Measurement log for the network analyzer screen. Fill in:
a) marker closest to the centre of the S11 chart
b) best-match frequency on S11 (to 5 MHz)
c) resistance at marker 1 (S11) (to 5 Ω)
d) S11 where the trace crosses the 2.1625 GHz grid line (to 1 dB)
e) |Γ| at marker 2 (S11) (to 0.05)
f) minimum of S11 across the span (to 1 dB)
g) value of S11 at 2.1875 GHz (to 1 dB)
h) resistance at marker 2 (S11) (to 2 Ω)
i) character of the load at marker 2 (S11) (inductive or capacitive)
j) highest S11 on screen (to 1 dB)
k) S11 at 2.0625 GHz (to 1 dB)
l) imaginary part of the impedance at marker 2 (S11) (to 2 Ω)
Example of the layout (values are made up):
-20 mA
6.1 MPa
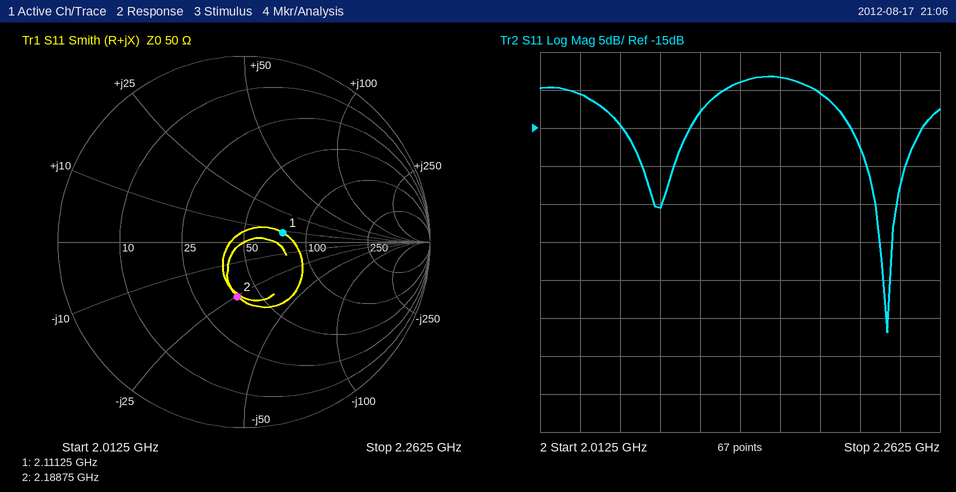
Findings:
marker 1
2.230 GHz
75 Ω
-8 dB
0.30
-42 dB
-10 dB
40 Ω
capacitive
-8 dB
-15 dB
-26 Ω
